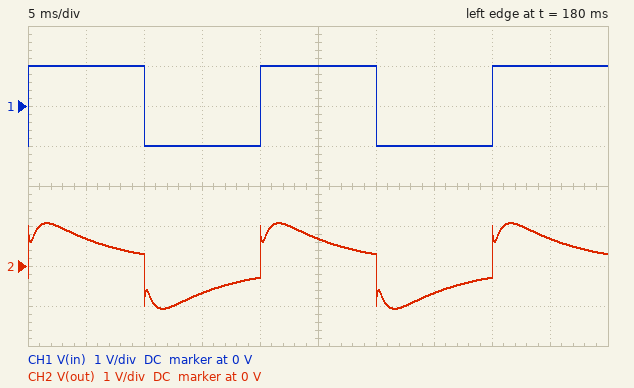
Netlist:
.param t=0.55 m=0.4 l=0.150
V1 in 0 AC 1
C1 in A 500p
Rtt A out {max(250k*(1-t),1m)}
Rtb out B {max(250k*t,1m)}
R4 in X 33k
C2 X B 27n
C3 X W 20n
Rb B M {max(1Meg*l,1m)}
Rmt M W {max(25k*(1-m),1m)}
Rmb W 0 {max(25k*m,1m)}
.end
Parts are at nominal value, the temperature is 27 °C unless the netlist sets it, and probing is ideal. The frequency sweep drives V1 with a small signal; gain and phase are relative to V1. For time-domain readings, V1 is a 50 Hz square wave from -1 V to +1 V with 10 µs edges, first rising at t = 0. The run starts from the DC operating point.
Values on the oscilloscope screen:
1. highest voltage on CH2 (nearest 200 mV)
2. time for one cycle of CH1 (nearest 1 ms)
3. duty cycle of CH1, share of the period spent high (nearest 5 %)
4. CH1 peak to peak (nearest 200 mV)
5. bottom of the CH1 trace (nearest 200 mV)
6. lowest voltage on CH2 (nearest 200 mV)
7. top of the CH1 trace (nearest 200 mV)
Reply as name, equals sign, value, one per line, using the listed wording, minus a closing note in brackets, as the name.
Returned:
highest voltage on CH2 = 1.0 V
time for one cycle of CH1 = 20 ms
duty cycle of CH1, share of the period spent high = 50 %
CH1 peak to peak = 2.0 V
bottom of the CH1 trace = -1.0 V
lowest voltage on CH2 = -1.0 V
top of the CH1 trace = 1.0 V
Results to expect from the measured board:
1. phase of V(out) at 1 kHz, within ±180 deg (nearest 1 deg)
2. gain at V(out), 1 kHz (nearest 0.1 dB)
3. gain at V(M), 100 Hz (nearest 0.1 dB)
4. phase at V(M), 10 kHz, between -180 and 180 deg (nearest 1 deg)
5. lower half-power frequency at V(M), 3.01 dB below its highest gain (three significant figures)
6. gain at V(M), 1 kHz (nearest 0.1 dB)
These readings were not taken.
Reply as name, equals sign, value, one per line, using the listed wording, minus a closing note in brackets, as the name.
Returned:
phase of V(out) at 1 kHz, within ±180 deg = 12 deg
gain at V(out), 1 kHz = -7.6 dB
gain at V(M), 100 Hz = -15.9 dB
phase at V(M), 10 kHz, between -180 and 180 deg = 1 deg
lower half-power frequency at V(M), 3.01 dB below its highest gain = 173 Hz
gain at V(M), 1 kHz = -12.5 dB
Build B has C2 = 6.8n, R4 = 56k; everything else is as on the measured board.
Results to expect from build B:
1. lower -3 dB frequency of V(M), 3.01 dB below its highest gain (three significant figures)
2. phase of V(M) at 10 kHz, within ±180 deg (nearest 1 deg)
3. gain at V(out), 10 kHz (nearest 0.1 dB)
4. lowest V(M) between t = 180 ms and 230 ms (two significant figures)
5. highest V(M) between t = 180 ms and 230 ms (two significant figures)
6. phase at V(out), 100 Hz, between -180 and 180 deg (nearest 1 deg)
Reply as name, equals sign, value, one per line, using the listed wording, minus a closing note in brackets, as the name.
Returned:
lower -3 dB frequency of V(M), 3.01 dB below its highest gain = 81.5 Hz
phase of V(M) at 10 kHz, within ±180 deg = 1 deg
gain at V(out), 10 kHz = -4.1 dB
lowest V(M) between t = 180 ms and 230 ms = -350 mV
highest V(M) between t = 180 ms and 230 ms = 350 mV
phase at V(out), 100 Hz, between -180 and 180 deg = 22 deg
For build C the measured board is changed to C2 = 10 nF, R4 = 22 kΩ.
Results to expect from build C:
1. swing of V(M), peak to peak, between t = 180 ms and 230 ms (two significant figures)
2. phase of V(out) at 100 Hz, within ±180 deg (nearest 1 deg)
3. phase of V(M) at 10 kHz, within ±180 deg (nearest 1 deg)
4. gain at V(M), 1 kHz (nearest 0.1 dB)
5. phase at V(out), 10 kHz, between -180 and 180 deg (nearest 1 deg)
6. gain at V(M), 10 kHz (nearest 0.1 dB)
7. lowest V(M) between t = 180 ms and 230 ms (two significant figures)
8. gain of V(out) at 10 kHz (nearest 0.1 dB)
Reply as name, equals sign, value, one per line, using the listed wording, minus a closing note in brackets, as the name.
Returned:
swing of V(M), peak to peak, between t = 180 ms and 230 ms = 1.3 V
phase of V(out) at 100 Hz, within ±180 deg = 26 deg
phase of V(M) at 10 kHz, within ±180 deg = 1 deg
gain at V(M), 1 kHz = -10.2 dB
phase at V(out), 10 kHz, between -180 and 180 deg = 3 deg
gain at V(M), 10 kHz = -9.6 dB
lowest V(M) between t = 180 ms and 230 ms = -650 mV
gain of V(out) at 10 kHz = -3.2 dB
